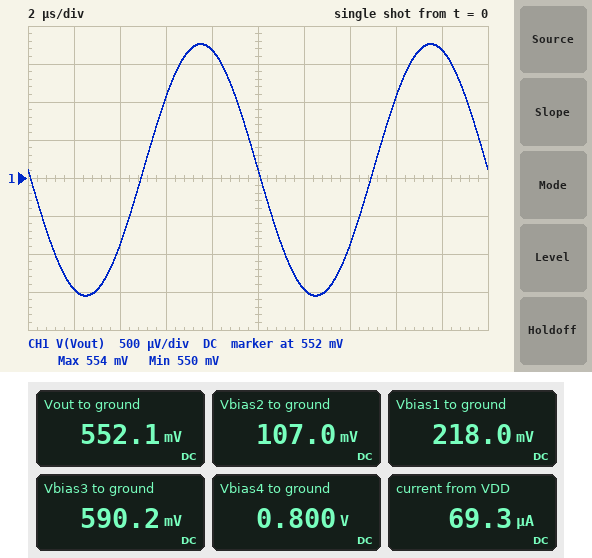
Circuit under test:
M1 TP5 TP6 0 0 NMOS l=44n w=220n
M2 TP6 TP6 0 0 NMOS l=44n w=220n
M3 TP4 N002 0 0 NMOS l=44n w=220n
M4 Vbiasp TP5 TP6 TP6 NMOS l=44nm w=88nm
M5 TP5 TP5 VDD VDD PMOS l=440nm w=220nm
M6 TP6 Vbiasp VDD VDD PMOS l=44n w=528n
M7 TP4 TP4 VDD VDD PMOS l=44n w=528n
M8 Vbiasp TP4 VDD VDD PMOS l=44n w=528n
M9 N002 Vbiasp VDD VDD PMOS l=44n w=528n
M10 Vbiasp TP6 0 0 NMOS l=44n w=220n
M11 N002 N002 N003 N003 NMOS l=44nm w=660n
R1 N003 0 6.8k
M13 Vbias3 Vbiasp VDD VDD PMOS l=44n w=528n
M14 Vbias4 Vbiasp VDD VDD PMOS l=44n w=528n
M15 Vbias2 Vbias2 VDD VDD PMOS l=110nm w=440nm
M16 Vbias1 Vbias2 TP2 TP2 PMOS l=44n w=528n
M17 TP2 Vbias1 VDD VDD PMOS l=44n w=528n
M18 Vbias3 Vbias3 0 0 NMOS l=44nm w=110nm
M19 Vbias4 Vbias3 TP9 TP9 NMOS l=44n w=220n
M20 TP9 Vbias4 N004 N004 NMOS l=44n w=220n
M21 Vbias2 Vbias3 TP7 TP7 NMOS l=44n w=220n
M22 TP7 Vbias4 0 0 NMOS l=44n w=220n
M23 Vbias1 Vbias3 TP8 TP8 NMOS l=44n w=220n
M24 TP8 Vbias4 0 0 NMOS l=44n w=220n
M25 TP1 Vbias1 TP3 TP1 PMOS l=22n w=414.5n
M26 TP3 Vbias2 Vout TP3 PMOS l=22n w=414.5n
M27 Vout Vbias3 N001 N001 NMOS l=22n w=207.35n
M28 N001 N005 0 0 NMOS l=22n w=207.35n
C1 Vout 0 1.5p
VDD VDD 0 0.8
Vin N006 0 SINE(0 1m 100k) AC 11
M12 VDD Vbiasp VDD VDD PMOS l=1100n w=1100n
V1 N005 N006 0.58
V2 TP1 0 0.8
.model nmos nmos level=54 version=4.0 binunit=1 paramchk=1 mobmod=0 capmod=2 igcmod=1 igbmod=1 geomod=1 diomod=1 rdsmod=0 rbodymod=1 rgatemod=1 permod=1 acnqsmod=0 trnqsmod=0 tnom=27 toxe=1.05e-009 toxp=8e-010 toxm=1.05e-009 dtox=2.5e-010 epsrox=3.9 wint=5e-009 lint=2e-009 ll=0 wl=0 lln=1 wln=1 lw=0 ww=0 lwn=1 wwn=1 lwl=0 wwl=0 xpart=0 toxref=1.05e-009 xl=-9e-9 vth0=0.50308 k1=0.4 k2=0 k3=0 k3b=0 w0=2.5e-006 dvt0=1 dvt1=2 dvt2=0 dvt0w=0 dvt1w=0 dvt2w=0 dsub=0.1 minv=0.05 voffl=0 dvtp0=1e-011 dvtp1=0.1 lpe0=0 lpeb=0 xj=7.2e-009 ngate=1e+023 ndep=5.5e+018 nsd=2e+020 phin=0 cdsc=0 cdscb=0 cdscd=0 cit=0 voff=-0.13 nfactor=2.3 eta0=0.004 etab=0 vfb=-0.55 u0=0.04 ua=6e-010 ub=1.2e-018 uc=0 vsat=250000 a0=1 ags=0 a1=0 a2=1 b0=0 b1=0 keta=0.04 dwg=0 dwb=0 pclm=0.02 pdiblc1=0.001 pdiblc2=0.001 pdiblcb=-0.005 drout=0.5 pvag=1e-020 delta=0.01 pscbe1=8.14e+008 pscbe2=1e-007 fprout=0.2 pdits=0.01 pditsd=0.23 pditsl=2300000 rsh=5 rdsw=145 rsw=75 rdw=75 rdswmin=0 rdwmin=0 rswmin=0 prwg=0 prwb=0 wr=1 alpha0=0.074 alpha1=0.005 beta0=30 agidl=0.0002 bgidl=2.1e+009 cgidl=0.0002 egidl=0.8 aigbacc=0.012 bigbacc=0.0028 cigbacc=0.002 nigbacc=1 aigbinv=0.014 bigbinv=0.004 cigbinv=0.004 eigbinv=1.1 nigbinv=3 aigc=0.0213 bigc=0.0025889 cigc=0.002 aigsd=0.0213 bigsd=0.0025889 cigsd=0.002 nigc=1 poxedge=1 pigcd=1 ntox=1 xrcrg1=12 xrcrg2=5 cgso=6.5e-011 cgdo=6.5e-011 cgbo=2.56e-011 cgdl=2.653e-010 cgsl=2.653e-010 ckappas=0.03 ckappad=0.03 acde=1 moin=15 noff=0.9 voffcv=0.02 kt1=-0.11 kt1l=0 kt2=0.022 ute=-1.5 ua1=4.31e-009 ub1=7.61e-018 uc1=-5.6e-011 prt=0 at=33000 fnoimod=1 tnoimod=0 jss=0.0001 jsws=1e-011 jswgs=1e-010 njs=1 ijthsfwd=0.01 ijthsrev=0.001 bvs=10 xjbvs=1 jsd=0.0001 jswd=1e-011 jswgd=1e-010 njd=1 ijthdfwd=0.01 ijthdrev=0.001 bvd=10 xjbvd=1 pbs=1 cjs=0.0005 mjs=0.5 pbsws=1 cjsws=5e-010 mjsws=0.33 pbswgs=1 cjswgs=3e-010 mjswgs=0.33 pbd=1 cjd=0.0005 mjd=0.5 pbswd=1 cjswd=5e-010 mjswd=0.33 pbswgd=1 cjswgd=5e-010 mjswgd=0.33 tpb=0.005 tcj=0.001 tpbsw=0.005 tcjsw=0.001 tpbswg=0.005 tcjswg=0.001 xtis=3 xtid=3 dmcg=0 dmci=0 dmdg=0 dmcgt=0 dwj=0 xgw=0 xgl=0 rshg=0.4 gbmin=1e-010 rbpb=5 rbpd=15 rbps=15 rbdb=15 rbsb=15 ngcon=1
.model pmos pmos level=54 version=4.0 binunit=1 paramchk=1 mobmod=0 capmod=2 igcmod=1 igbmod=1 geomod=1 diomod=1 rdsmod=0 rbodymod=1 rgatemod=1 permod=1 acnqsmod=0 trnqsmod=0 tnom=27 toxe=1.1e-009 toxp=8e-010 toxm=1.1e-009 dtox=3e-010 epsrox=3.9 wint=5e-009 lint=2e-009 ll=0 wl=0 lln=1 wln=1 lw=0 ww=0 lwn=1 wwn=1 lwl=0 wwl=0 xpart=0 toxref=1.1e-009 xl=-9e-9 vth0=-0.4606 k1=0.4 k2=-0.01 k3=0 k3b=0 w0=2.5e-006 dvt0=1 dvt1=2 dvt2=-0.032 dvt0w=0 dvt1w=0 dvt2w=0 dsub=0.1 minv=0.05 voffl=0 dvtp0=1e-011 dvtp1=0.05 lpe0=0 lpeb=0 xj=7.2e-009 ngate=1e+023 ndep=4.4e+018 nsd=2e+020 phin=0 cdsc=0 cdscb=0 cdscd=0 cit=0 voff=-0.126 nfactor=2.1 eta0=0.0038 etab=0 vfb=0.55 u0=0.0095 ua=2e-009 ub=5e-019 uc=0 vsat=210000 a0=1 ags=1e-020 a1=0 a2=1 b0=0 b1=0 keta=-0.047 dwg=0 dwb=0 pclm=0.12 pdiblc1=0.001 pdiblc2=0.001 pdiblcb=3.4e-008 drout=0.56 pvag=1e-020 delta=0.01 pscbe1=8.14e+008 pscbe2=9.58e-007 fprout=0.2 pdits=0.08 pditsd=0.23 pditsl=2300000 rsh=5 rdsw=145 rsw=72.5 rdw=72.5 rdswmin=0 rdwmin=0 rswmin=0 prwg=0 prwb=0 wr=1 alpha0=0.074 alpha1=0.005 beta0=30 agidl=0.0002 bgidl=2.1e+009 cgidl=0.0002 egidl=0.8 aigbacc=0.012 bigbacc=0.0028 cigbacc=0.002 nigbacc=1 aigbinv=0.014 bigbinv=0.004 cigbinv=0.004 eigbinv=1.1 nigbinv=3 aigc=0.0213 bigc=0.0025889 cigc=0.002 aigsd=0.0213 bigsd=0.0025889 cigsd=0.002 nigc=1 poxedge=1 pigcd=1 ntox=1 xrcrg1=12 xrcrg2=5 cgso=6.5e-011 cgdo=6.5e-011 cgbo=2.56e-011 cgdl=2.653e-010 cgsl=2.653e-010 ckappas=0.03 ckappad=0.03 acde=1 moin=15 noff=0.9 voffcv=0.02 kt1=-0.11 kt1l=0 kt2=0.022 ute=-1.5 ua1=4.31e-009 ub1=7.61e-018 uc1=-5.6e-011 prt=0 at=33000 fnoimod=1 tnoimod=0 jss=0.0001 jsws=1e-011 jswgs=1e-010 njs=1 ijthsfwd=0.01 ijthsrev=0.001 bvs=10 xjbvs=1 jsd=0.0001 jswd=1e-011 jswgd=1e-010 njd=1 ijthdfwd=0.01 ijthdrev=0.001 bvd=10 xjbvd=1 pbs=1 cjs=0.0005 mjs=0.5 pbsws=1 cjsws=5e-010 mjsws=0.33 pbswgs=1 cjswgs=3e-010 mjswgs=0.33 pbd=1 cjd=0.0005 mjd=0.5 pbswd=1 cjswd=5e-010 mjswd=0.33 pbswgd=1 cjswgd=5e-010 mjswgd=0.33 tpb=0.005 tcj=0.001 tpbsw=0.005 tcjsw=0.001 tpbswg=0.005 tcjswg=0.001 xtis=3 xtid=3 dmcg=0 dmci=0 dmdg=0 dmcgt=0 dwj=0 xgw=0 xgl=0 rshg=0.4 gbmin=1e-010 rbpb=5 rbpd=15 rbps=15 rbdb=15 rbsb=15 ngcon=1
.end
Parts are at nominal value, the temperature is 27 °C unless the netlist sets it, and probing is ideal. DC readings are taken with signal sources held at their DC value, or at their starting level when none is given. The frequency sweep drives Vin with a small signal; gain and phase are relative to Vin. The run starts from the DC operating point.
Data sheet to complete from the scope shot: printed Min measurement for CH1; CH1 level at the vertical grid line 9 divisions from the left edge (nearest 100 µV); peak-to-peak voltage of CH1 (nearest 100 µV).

550 mV
553.7 mV
3.3 mV
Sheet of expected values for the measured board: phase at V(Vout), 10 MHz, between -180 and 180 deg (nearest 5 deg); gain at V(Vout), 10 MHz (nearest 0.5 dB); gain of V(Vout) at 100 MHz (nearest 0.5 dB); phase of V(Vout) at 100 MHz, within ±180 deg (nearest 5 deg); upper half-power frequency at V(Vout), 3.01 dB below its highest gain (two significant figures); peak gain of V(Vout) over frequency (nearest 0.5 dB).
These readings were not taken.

145 deg
2.5 dB
-13.0 dB
100 deg
14 MHz
4.5 dB
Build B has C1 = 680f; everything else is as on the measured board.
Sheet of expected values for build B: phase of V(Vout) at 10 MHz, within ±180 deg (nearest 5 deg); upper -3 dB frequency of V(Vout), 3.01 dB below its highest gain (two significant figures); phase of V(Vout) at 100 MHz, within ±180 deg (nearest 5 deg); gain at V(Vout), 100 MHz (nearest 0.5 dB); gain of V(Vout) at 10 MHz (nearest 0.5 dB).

160 deg
31 MHz
105 deg
-6.5 dB
4.0 dB
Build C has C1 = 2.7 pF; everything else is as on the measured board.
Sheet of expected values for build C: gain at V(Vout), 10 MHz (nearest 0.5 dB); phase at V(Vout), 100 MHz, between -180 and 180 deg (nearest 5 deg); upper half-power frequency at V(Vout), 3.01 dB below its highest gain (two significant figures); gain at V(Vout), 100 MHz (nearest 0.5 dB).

0 dB
95 deg
7.7 MHz
-18.0 dB
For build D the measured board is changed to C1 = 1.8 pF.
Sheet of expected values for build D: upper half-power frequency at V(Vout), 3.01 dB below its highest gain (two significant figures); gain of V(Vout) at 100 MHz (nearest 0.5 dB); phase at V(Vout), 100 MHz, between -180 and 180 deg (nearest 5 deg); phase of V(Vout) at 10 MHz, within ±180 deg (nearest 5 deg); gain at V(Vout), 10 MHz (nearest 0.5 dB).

12 MHz
-14.5 dB
95 deg
140 deg
2.0 dB
